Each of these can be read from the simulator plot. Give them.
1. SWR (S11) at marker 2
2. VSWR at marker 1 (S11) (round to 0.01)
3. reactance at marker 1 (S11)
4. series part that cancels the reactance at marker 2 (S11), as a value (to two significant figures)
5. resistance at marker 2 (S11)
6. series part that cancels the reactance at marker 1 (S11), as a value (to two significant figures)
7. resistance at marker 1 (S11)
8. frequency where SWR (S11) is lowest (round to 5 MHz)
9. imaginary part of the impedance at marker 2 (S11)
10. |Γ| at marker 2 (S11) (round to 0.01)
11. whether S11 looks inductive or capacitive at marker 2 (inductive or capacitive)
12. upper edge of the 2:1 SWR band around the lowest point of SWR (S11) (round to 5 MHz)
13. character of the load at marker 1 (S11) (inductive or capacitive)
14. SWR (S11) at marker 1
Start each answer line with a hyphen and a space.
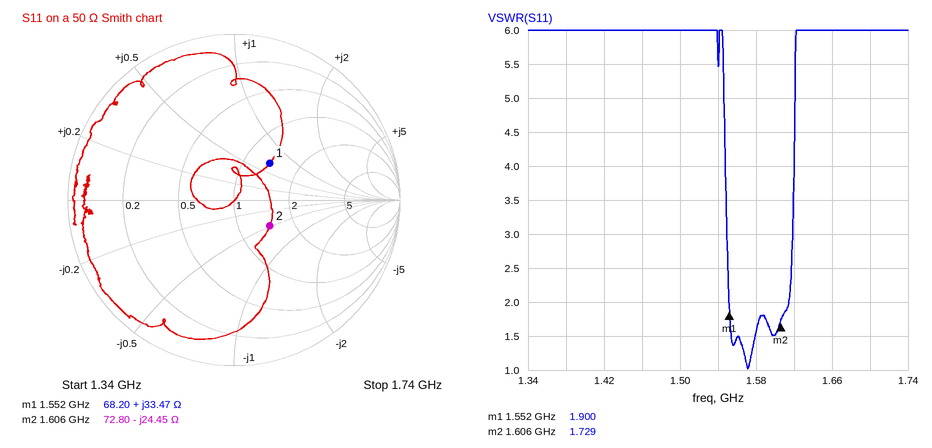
- 1.729
- 1.90
- +33.47 Ω
- 2.4 nH
- 72.80 Ω
- 3.1 pF
- 68.20 Ω
- 1.570 GHz
- -24.45 Ω
- 0.27
- capacitive
- 1.615 GHz
- inductive
- 1.900
